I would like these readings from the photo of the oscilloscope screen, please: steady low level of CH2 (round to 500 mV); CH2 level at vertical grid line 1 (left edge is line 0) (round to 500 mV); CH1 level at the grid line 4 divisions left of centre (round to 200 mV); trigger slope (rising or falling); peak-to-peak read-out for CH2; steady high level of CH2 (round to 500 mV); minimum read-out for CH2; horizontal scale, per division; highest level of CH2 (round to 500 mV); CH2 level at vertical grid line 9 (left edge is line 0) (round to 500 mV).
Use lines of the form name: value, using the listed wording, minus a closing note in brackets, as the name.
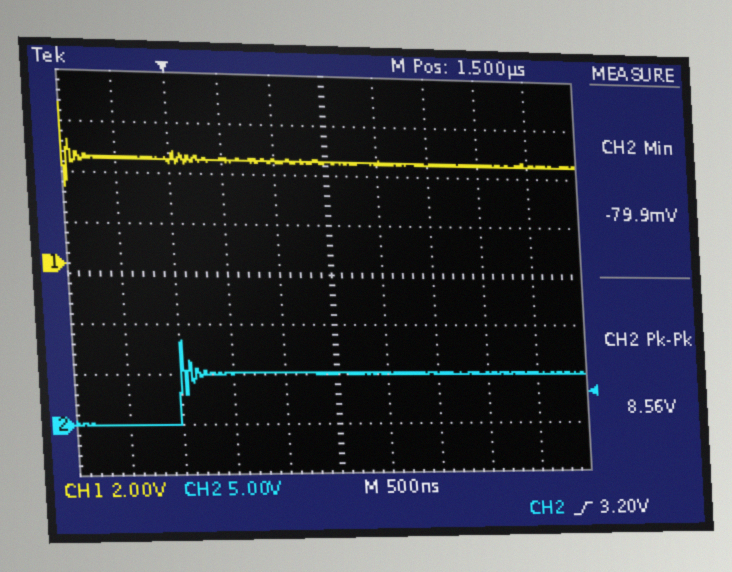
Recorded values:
steady low level of CH2: 0.0 V
CH2 level at vertical grid line 1 (left edge is line 0): 0.0 V
CH1 level at the grid line 4 divisions left of centre: 4.2 V
trigger slope: rising
peak-to-peak read-out for CH2: 8.56 V
steady high level of CH2: 5.0 V
minimum read-out for CH2: -79.9 mV
horizontal scale, per division: 500 ns
highest level of CH2: 8.5 V
CH2 level at vertical grid line 9 (left edge is line 0): 5.0 V
